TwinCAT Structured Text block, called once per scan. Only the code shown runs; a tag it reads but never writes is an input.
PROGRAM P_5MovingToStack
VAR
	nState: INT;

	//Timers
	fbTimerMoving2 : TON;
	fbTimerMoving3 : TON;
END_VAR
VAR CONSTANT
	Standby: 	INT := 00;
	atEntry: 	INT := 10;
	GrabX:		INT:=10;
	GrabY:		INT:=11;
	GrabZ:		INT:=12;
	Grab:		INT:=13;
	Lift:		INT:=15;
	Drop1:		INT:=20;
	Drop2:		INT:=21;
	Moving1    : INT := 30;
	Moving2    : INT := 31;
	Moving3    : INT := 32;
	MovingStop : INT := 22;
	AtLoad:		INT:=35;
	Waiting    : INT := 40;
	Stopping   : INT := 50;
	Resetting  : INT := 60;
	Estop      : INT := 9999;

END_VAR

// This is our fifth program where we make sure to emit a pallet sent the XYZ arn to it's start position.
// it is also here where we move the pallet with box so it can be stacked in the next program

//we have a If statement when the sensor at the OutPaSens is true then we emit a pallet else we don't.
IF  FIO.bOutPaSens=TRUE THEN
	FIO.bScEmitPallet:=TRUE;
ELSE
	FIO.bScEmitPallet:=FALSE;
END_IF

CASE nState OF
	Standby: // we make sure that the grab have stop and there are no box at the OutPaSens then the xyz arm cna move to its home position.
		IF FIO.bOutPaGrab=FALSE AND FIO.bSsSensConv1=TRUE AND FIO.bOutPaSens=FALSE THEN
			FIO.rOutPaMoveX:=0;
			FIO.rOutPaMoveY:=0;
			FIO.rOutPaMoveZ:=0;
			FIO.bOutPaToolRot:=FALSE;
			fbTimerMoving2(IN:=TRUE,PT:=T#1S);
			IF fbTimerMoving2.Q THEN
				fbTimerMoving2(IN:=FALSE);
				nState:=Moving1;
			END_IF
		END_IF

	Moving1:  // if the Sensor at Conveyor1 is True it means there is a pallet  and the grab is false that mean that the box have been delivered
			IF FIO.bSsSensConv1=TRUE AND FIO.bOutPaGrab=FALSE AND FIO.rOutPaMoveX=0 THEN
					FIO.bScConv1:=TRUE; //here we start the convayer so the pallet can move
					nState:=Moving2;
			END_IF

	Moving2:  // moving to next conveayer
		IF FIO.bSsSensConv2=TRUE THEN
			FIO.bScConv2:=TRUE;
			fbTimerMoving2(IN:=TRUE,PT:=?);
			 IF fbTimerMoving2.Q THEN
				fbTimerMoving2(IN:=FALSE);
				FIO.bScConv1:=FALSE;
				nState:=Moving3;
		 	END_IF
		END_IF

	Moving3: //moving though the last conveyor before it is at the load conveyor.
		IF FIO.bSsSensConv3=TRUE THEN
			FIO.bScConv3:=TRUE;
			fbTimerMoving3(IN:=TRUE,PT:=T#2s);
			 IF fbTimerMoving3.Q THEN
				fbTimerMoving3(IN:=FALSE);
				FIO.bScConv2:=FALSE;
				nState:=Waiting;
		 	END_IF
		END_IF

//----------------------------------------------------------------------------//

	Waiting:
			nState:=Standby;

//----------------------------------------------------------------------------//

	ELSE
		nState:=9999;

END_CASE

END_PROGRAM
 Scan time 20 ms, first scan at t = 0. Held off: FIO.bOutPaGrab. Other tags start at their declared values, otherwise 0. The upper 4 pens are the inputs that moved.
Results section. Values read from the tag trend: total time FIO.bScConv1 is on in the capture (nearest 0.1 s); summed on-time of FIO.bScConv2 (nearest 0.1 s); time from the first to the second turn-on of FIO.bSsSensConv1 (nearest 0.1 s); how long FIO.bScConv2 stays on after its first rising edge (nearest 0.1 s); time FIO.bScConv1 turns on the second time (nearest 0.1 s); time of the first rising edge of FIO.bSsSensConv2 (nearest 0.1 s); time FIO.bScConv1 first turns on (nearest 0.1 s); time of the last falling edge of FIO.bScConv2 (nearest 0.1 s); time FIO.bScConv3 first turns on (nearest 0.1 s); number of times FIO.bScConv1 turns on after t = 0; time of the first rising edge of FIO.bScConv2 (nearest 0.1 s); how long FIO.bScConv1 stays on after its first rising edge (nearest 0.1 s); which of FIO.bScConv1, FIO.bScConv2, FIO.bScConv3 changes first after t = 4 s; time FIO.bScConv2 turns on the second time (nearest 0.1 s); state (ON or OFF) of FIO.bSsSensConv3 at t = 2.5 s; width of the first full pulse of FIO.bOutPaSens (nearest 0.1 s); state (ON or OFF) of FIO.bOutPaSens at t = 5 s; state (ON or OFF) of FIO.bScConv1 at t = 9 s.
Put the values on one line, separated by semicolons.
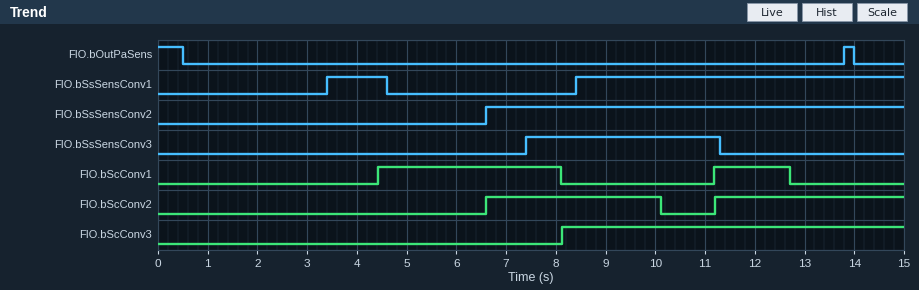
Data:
5.2 s; 7.3 s; 5.0 s; 3.5 s; 11.2 s; 6.6 s; 4.4 s; 10.1 s; 8.1 s; 2; 6.6 s; 3.7 s; FIO.bScConv1; 11.2 s; OFF; 0.2 s; OFF; OFF
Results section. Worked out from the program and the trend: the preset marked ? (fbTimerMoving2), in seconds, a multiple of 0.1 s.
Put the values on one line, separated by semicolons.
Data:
1.5 s
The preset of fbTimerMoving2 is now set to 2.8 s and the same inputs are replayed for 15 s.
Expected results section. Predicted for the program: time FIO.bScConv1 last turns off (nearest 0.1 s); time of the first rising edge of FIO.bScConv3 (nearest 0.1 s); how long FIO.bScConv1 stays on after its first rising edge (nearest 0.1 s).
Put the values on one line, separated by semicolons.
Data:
9.4 s; 9.4 s; 5.0 s
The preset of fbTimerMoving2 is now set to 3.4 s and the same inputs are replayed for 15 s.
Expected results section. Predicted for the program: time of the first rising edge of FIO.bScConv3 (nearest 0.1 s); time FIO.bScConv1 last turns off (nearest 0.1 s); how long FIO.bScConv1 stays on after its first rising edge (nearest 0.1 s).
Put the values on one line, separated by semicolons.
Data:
10.0 s; 10.0 s; 5.6 s
